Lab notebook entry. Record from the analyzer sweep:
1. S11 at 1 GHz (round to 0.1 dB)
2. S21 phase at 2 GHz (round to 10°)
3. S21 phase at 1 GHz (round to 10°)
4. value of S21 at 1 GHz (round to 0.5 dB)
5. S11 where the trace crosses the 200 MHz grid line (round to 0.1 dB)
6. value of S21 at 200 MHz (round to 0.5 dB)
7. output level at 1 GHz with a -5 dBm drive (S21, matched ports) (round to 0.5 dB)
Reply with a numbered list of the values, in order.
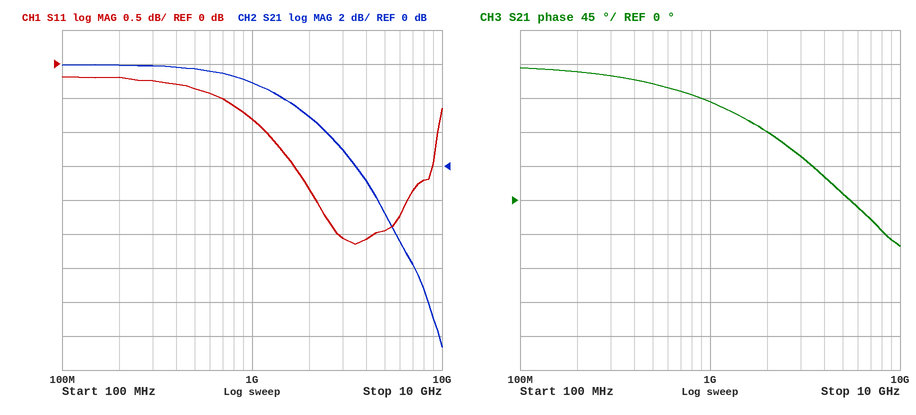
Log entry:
1. -0.8 dB
2. 90°
3. 130°
4. 5.0 dB
5. -0.2 dB
6. 6.0 dB
7. 0.0 dBm
